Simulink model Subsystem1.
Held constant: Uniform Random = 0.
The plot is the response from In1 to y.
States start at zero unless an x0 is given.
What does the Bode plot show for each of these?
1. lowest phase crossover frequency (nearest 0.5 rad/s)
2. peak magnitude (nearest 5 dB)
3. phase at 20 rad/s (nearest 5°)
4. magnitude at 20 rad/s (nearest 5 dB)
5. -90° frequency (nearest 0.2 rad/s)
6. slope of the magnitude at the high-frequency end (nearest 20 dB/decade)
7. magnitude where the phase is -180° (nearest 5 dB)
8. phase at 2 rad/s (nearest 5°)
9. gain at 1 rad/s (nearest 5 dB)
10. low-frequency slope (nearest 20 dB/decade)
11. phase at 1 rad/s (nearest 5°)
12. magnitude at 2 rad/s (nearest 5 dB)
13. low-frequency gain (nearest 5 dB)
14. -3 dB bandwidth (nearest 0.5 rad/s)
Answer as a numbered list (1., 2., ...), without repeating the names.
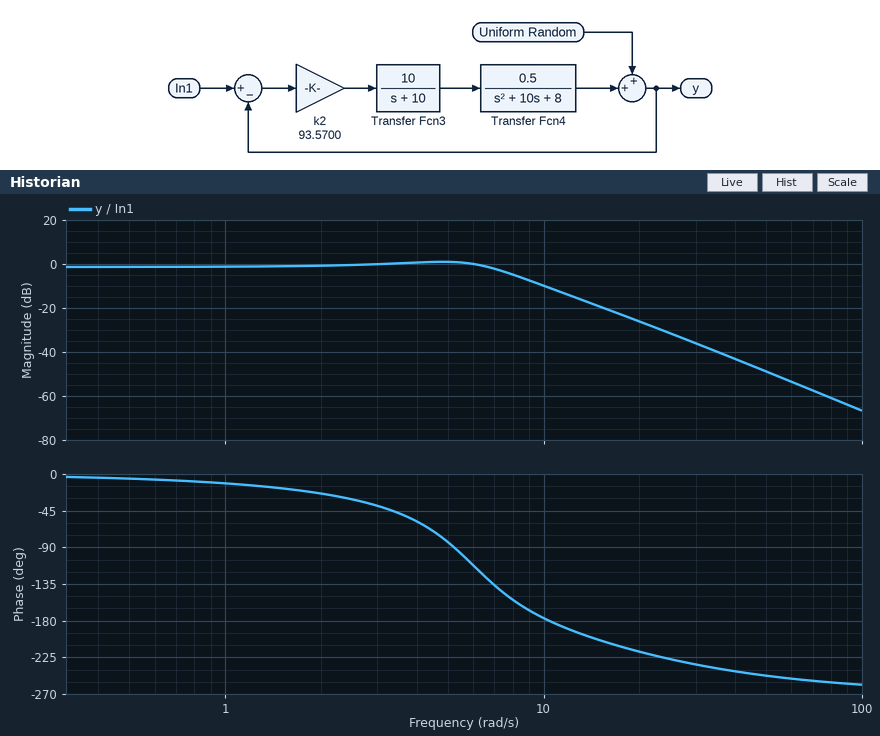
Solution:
1. 10.5 rad/s
2. 0 dB
3. -220°
4. -25 dB
5. 5.2 rad/s
6. -60 dB/decade
7. -10 dB
8. -25°
9. 0 dB
10. 0 dB/decade
11. -10°
12. 0 dB
13. 0 dB
14. 8.0 rad/s
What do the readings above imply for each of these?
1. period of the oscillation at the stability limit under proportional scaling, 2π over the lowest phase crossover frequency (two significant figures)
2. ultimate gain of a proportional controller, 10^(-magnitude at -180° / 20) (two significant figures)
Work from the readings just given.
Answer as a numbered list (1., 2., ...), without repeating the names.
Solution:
1. 0.60 s
2. 3.2
